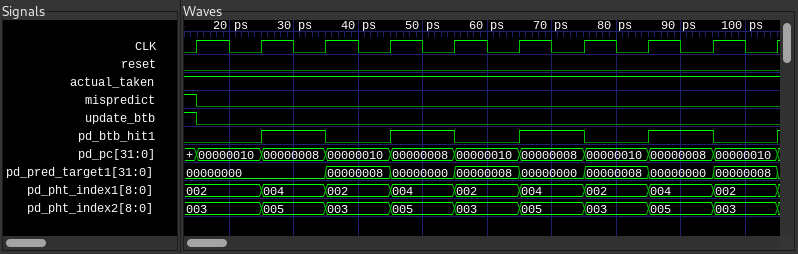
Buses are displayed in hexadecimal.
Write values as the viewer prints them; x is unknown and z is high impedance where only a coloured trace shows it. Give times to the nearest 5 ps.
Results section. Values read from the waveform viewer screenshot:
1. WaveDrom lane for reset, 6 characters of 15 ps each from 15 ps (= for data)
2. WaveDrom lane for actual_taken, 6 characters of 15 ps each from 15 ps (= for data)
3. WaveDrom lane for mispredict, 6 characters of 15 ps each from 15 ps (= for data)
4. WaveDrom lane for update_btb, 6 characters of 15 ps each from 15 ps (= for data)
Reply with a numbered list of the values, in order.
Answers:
1. {name: 'reset', wave: '0.....'}
2. {name: 'actual_taken', wave: '1.....'}
3. {name: 'mispredict', wave: '0.....'}
4. {name: 'update_btb', wave: '0.....'}
